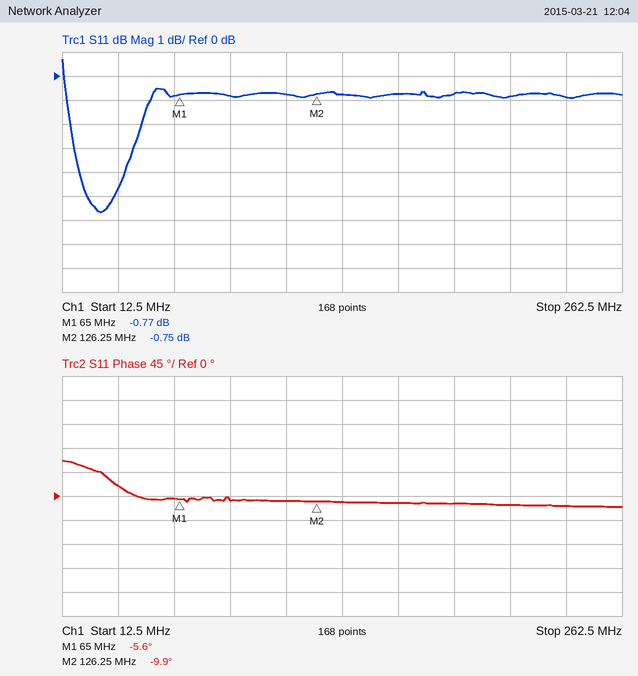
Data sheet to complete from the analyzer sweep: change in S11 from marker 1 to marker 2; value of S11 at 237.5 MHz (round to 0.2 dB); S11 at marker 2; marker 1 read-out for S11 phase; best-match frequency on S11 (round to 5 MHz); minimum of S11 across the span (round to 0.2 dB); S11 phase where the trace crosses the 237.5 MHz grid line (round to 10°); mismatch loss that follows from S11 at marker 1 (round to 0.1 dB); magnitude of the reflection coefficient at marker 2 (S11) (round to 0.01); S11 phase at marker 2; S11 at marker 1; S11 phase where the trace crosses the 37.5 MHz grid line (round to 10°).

0.02 dB
-0.8 dB
-0.75 dB
-5.6°
30 MHz
-5.6 dB
-20°
7.9 dB
0.92
-9.9°
-0.77 dB
20°
